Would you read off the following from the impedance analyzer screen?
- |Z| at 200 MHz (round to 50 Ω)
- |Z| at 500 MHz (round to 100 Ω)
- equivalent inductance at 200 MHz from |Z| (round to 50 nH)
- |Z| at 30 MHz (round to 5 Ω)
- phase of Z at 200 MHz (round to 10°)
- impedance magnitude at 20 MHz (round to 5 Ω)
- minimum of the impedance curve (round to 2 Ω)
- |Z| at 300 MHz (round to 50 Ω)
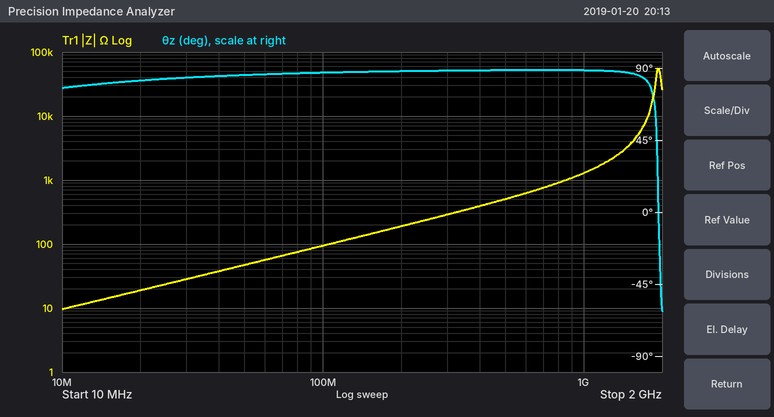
200 Ω
500 Ω
150 nH
30 Ω
90°
20 Ω
10 Ω
300 Ω
